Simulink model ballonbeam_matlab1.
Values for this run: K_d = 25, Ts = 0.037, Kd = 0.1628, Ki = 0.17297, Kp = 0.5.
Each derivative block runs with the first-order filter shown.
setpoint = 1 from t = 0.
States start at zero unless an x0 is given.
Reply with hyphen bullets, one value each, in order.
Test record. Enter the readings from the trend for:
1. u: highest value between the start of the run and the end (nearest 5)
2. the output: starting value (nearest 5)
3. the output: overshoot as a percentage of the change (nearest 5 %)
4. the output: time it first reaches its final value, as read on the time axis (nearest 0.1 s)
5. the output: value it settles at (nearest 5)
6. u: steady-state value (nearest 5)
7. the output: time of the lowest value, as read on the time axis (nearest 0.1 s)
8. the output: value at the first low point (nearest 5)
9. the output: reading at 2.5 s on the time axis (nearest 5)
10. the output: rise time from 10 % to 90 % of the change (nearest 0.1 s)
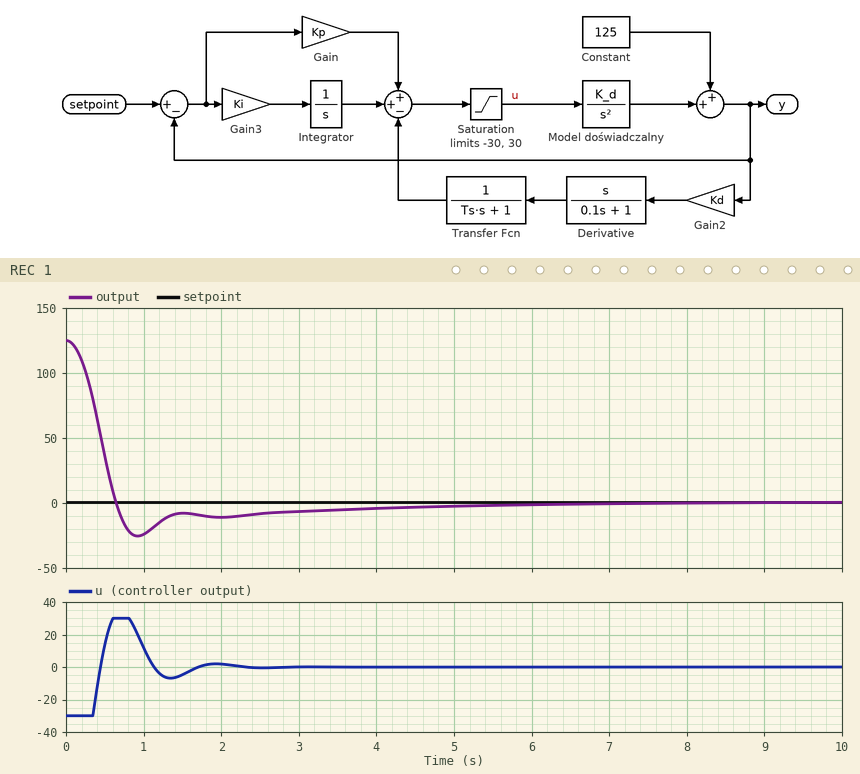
- 30
- 125
- 20 %
- 0.6 s
- 0
- 0
- 0.9 s
- -25
- -10
- 0.4 s
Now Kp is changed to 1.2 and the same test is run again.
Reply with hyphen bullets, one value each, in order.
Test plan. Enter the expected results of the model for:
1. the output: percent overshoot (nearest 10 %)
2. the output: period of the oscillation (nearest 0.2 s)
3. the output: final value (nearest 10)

- 50 %
- 1.2 s
- 0
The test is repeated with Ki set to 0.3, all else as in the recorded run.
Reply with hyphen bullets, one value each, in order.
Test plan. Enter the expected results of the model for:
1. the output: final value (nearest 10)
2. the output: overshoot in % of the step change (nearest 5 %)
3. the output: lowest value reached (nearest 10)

- 0
- 30 %
- -40
